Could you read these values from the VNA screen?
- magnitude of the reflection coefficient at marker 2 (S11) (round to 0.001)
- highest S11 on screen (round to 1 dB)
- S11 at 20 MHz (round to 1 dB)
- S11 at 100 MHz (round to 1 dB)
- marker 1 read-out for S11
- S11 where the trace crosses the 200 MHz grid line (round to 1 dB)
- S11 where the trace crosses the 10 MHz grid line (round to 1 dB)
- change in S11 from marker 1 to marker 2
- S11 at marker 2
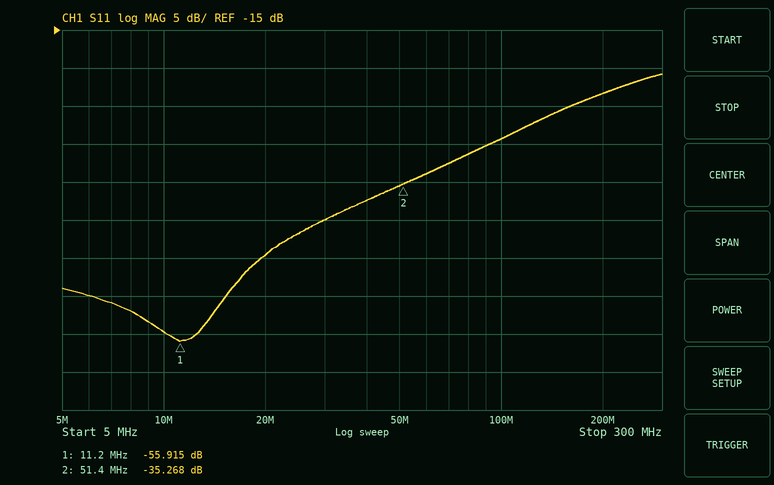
0.017
-21 dB
-45 dB
-29 dB
-55.915 dB
-23 dB
-55 dB
20.647 dB
-35.268 dB
